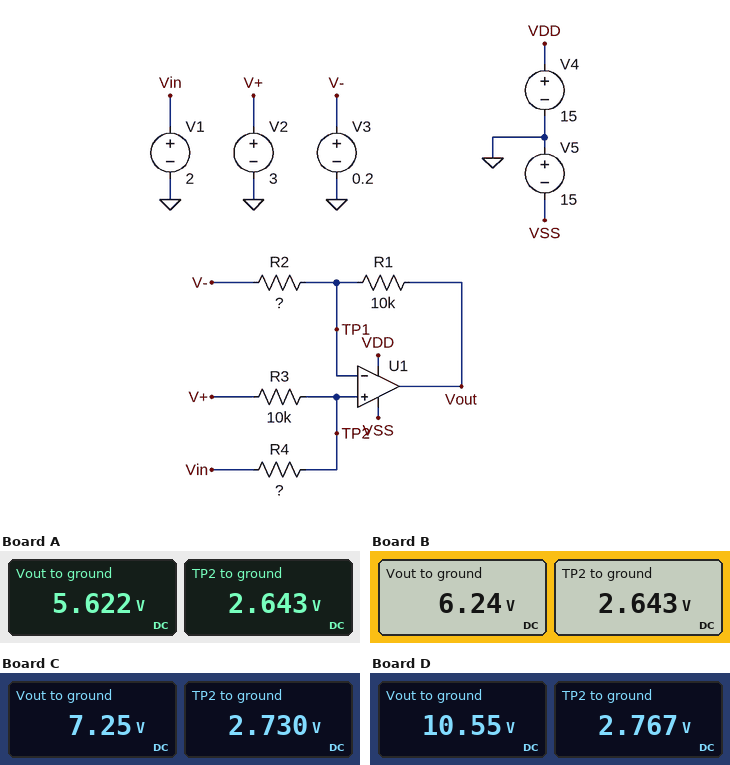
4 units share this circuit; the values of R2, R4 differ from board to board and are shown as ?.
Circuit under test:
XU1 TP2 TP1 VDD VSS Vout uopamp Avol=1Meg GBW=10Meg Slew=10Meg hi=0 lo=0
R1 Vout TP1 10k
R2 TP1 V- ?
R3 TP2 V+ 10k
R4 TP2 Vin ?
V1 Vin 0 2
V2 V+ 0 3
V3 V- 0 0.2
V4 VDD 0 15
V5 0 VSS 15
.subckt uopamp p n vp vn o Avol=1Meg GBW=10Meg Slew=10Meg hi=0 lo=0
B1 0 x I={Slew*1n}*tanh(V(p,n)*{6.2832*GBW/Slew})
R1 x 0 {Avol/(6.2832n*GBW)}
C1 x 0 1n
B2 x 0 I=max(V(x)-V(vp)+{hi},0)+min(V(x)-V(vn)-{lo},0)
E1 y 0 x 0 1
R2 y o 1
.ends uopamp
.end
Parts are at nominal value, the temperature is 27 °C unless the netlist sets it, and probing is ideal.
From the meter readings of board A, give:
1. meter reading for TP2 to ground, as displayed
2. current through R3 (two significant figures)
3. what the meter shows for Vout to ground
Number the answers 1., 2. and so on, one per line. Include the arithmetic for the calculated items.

1. 2.643 V
2. (3 V - 2.643 V) / 10 kΩ = 36 µA
3. 5.622 V
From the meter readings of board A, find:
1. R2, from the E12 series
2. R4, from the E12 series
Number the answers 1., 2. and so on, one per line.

1. 8.2 kΩ
2. 18 kΩ
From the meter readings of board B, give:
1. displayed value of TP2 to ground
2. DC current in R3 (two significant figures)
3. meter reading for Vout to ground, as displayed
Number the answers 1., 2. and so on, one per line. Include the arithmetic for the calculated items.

1. 2.643 V
2. (3 V - 2.643 V) / 10 kΩ = 36 µA
3. 6.24 V
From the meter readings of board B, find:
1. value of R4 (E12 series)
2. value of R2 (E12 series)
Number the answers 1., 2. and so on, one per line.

1. 18 kΩ
2. 6.8 kΩ
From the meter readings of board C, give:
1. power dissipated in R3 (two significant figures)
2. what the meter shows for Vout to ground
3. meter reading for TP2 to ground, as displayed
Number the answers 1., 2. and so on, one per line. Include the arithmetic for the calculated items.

1. (3 V - 2.73 V)^2 / 10 kΩ = 7.3 µW
2. 7.25 V
3. 2.730 V
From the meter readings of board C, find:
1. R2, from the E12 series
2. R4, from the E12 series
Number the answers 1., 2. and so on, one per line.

1. 5.6 kΩ
2. 27 kΩ
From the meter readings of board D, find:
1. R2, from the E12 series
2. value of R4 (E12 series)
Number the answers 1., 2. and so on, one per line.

1. 3.3 kΩ
2. 33 kΩ
